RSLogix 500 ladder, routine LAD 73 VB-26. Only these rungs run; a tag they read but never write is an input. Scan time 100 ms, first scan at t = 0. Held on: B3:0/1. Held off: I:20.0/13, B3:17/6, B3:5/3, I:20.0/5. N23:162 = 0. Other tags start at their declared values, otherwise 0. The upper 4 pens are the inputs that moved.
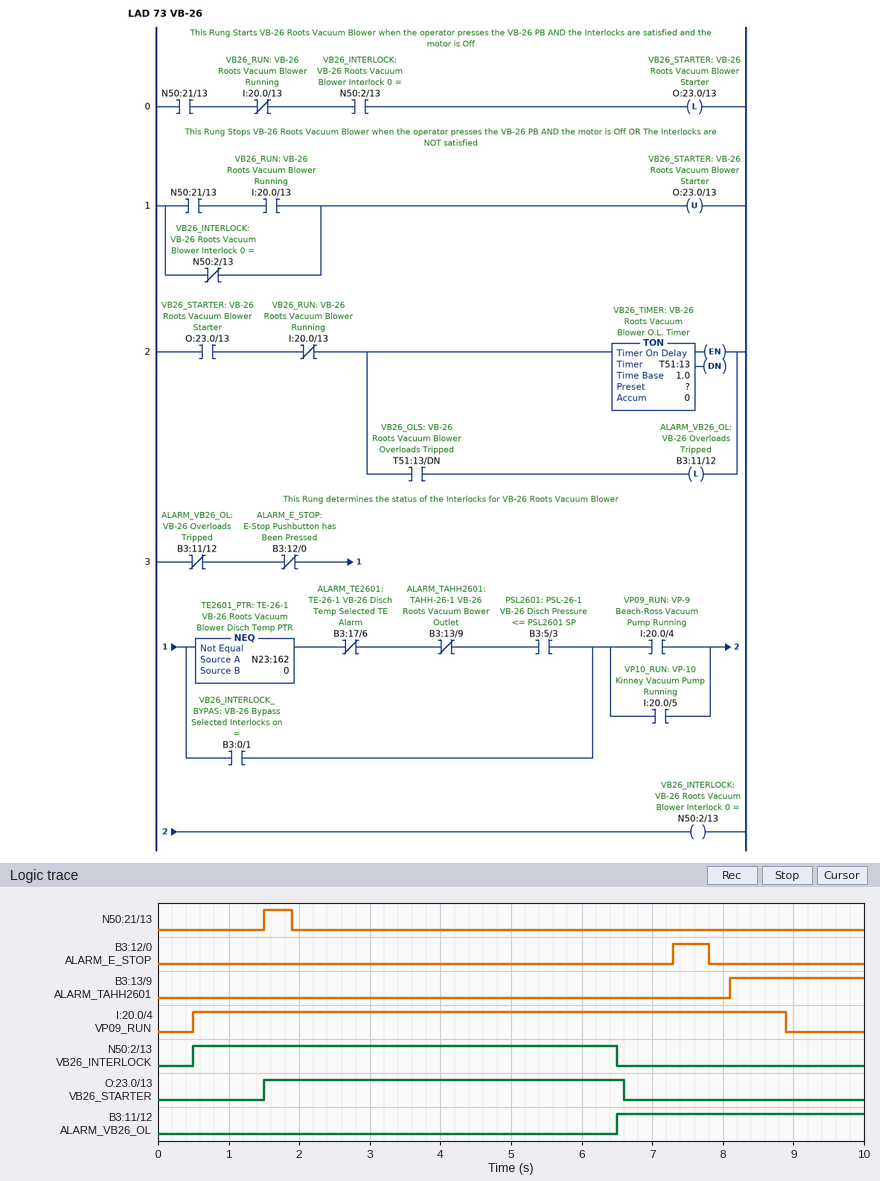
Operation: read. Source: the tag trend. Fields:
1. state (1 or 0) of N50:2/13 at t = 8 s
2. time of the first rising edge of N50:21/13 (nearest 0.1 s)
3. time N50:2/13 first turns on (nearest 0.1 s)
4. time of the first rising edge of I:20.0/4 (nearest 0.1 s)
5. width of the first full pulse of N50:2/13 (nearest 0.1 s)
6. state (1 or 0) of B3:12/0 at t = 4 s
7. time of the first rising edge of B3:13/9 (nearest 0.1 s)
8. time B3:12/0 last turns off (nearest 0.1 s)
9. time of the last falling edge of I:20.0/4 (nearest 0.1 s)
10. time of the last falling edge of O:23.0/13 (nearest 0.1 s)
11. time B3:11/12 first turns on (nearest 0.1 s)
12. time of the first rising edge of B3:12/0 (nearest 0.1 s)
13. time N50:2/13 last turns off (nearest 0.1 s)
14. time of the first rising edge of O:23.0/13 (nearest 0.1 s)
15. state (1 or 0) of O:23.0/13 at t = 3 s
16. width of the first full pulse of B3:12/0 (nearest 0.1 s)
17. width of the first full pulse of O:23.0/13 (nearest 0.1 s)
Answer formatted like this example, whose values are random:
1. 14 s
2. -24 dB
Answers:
1. 0
2. 1.5 s
3. 0.5 s
4. 0.5 s
5. 6.0 s
6. 0
7. 8.1 s
8. 7.8 s
9. 8.9 s
10. 6.6 s
11. 6.5 s
12. 7.3 s
13. 6.5 s
14. 1.5 s
15. 1
16. 0.5 s
17. 5.1 s
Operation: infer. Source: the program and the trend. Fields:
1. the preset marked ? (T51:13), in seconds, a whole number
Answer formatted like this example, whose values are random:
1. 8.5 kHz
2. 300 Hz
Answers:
1. 5 s
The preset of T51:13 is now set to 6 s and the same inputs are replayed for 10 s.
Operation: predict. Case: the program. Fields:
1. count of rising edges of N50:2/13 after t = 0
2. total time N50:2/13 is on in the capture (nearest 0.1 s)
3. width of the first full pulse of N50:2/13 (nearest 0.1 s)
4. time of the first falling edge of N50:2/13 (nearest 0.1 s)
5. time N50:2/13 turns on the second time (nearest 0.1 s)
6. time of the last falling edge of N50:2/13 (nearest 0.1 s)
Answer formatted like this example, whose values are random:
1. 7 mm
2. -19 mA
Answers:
1. 2
2. 7.9 s
3. 6.8 s
4. 7.3 s
5. 7.8 s
6. 8.9 s
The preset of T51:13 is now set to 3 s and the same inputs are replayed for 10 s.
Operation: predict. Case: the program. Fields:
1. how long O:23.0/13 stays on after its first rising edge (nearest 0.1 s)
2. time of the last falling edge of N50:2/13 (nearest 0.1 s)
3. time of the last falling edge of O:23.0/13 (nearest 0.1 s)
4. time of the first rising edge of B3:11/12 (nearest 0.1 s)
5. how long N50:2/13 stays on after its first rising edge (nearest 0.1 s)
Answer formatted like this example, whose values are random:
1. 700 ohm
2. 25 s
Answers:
1. 3.1 s
2. 4.5 s
3. 4.6 s
4. 4.5 s
5. 4.0 s
